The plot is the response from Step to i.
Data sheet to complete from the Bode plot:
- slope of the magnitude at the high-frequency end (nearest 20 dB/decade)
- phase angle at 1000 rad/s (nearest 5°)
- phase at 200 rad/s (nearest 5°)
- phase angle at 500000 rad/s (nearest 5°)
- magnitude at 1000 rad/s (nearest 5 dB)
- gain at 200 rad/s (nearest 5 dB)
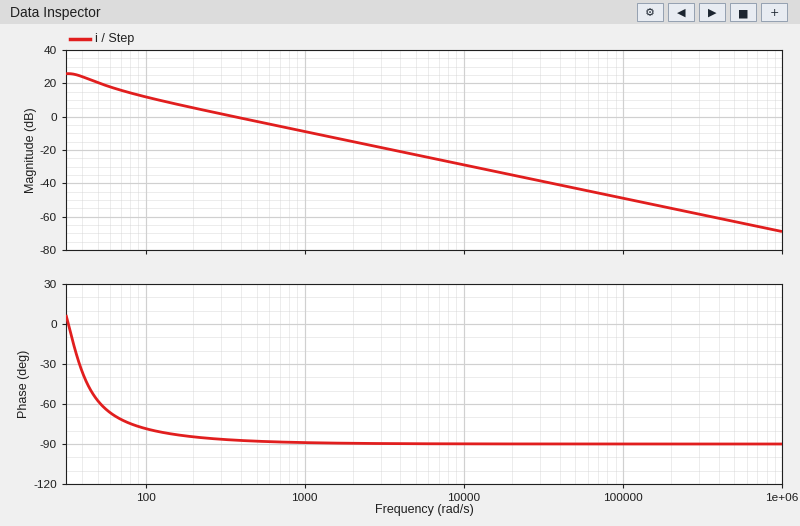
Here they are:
-20 dB/decade
-90°
-85°
-90°
-10 dB
5 dB
